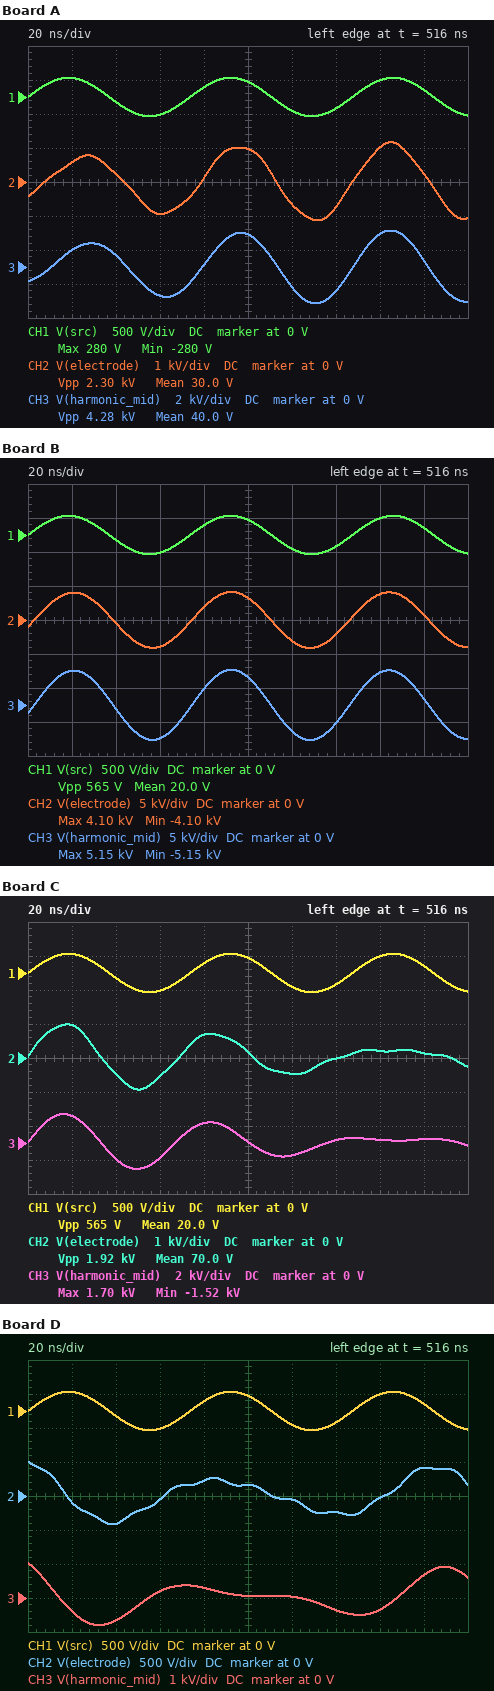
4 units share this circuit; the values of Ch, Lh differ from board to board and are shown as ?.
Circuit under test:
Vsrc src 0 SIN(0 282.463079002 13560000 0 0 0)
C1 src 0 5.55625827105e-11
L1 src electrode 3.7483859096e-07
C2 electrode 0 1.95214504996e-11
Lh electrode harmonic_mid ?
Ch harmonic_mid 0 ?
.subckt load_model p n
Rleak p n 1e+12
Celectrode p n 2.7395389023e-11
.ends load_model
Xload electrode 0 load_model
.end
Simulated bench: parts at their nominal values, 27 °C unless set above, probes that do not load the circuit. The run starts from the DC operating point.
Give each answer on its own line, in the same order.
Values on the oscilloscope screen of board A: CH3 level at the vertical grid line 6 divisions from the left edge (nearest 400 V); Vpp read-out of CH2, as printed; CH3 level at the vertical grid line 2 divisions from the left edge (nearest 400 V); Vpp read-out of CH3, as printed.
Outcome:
-1.2 kV
2.30 kV
800 V
4.28 kV
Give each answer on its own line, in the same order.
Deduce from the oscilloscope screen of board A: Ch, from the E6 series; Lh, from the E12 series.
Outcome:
100 pF
560 nH
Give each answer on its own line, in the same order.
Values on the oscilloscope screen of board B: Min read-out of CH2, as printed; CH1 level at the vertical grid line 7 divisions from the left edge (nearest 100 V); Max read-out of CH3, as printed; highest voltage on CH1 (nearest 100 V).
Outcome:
-4.10 kV
-200 V
5.15 kV
300 V
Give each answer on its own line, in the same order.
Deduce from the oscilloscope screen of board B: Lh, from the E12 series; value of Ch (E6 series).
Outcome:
120 nH
220 pF
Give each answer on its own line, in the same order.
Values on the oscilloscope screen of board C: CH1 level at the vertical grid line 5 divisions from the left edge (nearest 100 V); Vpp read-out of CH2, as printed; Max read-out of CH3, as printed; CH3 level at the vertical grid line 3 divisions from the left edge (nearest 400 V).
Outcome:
200 V
1.92 kV
1.70 kV
-800 V
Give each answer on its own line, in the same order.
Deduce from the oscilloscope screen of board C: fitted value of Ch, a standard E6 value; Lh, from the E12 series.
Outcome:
100 pF
470 nH
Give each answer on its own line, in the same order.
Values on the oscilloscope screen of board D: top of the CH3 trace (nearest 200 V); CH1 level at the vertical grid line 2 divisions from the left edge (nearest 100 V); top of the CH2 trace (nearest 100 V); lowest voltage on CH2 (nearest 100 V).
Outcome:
1.0 kV
-100 V
500 V
-400 V
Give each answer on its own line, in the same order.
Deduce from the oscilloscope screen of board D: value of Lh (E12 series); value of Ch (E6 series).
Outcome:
390 nH
220 pF
